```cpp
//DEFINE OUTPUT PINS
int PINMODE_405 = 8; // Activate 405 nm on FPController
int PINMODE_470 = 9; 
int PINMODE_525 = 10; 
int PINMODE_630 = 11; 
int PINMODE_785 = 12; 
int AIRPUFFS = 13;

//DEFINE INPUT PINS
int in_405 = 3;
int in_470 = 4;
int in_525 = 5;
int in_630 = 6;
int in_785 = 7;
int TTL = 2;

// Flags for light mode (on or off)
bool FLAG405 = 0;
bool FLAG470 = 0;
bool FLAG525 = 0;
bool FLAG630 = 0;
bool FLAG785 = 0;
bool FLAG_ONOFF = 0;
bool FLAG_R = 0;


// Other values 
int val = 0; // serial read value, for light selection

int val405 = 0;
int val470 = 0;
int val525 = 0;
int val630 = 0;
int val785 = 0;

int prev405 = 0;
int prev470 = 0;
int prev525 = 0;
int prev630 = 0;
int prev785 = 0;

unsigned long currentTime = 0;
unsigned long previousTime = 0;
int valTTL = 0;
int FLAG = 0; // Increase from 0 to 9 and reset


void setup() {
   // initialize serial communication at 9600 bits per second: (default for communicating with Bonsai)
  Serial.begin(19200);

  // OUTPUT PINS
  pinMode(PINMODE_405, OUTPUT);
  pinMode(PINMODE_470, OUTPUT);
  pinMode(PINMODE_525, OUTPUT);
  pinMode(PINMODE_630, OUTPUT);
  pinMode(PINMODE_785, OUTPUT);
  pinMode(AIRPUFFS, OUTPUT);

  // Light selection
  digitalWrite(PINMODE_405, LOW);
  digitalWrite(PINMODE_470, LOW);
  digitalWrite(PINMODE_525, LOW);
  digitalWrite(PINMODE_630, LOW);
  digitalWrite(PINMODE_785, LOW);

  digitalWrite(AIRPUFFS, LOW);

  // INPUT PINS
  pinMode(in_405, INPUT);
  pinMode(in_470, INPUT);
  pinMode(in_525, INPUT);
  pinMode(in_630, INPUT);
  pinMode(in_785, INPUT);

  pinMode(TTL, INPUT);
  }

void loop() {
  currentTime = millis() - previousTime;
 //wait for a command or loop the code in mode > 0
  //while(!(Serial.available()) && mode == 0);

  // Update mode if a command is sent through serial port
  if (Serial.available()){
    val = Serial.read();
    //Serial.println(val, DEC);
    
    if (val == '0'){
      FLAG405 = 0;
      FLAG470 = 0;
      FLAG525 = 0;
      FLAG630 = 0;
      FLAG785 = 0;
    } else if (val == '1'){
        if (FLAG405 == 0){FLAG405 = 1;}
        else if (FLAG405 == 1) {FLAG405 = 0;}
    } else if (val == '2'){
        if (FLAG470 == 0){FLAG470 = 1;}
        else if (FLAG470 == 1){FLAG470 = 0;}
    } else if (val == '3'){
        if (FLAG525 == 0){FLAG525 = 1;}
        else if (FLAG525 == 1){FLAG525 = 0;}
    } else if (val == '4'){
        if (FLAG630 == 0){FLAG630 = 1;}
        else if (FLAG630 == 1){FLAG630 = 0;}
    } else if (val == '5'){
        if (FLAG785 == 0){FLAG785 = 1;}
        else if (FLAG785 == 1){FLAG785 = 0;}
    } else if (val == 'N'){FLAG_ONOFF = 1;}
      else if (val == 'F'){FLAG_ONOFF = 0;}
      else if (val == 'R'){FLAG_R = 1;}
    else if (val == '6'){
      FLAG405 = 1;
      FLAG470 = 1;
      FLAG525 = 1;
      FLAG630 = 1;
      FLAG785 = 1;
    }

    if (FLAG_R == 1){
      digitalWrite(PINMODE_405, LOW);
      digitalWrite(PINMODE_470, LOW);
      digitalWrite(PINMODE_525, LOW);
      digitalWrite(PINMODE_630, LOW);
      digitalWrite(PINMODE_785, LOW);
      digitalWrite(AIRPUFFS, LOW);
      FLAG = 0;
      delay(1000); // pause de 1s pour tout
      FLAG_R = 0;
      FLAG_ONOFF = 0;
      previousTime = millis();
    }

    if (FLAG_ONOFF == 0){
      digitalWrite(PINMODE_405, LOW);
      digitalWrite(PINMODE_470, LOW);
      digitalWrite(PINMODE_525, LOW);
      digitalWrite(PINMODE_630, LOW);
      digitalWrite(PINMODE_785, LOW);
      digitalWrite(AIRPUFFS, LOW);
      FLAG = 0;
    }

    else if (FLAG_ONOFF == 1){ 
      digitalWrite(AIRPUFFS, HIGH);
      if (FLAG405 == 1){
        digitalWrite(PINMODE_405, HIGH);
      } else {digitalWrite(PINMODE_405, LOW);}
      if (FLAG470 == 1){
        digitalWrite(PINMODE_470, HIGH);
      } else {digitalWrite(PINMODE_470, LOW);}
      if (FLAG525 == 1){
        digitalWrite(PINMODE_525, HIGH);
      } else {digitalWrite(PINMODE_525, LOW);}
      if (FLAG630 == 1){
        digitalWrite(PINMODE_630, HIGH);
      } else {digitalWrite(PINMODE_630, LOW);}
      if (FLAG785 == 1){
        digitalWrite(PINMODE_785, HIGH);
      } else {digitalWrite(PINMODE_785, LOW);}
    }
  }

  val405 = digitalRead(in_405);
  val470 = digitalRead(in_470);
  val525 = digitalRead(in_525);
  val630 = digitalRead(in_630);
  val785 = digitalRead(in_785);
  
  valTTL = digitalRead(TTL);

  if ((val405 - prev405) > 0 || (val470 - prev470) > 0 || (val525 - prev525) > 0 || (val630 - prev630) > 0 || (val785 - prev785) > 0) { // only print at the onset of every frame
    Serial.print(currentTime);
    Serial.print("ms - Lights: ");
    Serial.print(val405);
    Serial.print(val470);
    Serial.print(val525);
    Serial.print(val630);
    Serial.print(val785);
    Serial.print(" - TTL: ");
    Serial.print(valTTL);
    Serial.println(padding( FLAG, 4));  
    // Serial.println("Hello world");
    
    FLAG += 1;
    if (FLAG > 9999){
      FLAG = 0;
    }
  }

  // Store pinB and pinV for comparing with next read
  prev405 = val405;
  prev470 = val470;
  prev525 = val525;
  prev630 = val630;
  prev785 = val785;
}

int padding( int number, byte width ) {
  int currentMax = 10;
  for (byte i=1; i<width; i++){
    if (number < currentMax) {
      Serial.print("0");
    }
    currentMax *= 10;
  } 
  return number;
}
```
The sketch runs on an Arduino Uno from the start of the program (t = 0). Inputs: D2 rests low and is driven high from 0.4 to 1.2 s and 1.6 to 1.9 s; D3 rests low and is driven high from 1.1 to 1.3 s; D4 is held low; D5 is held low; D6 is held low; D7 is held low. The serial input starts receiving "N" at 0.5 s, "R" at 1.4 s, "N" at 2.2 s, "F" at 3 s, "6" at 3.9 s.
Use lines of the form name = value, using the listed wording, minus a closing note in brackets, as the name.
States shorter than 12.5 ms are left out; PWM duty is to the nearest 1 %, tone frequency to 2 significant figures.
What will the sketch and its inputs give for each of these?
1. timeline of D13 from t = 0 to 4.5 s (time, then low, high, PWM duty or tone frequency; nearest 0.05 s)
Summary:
timeline of D13 from t = 0 to 4.5 s = 0 s low; 0.5 s high; 1.4 s low; 2.4 s high; 3 s low
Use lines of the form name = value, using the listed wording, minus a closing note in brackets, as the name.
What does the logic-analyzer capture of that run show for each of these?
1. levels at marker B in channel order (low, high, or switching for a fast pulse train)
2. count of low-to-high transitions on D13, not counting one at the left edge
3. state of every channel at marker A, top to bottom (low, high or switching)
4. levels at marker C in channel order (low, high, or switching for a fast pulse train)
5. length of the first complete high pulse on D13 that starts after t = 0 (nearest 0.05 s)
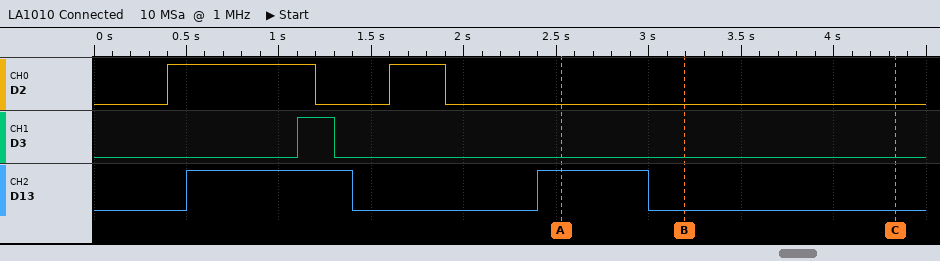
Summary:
levels at marker B in channel order = D2 low, D3 low, D13 low
count of low-to-high transitions on D13, not counting one at the left edge = 2
state of every channel at marker A, top to bottom = D2 low, D3 low, D13 high
levels at marker C in channel order = D2 low, D3 low, D13 low
length of the first complete high pulse on D13 that starts after t = 0 = 0.90 s
